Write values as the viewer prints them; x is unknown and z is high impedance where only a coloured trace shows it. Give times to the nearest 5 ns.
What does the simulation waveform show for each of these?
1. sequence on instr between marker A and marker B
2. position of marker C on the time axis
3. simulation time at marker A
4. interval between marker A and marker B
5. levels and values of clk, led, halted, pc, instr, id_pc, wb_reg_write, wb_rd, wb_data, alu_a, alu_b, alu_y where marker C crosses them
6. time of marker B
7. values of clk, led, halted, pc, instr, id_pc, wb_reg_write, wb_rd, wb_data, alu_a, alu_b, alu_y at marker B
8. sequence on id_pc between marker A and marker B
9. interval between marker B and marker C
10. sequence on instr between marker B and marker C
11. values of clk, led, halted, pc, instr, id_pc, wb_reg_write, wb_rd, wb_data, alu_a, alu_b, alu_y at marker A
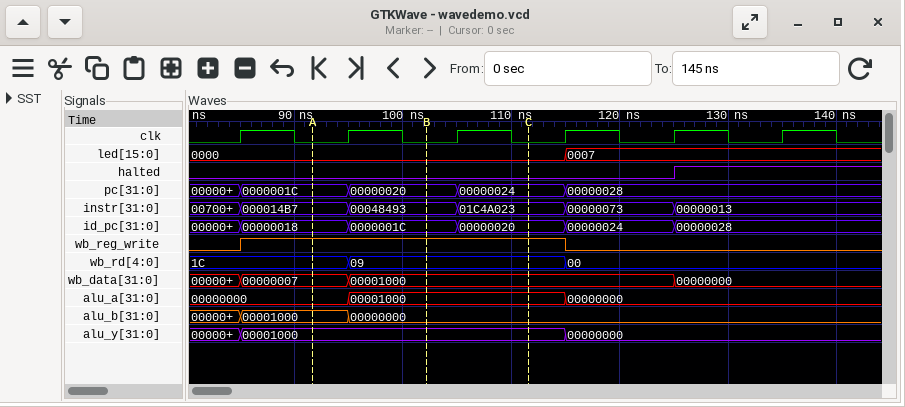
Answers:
000014B7, 00048493
110 ns
90 ns
10 ns
clk=0, led=0000, halted=0, pc=00000024, instr=01C4A023, id_pc=00000020, wb_reg_write=1, wb_rd=09, wb_data=00001000, alu_a=00001000, alu_b=00000000, alu_y=00001000
100 ns
clk=0, led=0000, halted=0, pc=00000020, instr=00048493, id_pc=0000001C, wb_reg_write=1, wb_rd=09, wb_data=00001000, alu_a=00001000, alu_b=00000000, alu_y=00001000
00000018, 0000001C
10 ns
00048493, 01C4A023
clk=0, led=0000, halted=0, pc=0000001C, instr=000014B7, id_pc=00000018, wb_reg_write=1, wb_rd=1C, wb_data=00000007, alu_a=00000000, alu_b=00001000, alu_y=00001000
